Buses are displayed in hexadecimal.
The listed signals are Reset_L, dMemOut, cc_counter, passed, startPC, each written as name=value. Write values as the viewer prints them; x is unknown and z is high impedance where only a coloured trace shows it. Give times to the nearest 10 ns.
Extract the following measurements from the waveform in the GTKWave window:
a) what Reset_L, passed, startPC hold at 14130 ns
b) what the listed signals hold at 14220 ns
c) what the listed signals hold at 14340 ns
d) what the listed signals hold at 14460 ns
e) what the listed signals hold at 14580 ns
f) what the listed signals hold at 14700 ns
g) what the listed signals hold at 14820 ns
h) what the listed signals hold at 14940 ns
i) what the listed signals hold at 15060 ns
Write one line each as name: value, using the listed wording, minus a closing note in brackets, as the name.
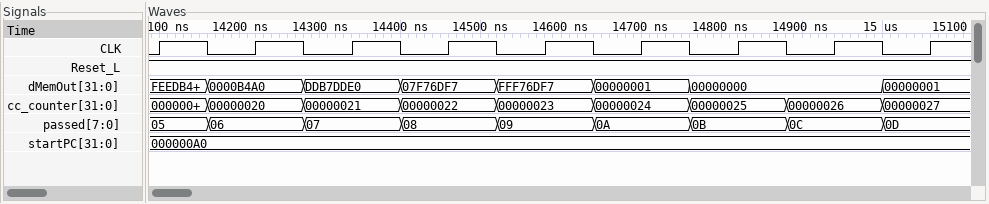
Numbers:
what Reset_L, passed, startPC hold at 14130 ns: Reset_L=1, passed=05, startPC=000000A0
what the listed signals hold at 14220 ns: Reset_L=1, dMemOut=0000B4A0, cc_counter=00000020, passed=06, startPC=000000A0
what the listed signals hold at 14340 ns: Reset_L=1, dMemOut=DDB7DDE0, cc_counter=00000021, passed=07, startPC=000000A0
what the listed signals hold at 14460 ns: Reset_L=1, dMemOut=07F76DF7, cc_counter=00000022, passed=08, startPC=000000A0
what the listed signals hold at 14580 ns: Reset_L=1, dMemOut=FFF76DF7, cc_counter=00000023, passed=09, startPC=000000A0
what the listed signals hold at 14700 ns: Reset_L=1, dMemOut=00000001, cc_counter=00000024, passed=0A, startPC=000000A0
what the listed signals hold at 14820 ns: Reset_L=1, dMemOut=00000000, cc_counter=00000025, passed=0B, startPC=000000A0
what the listed signals hold at 14940 ns: Reset_L=1, dMemOut=00000000, cc_counter=00000026, passed=0C, startPC=000000A0
what the listed signals hold at 15060 ns: Reset_L=1, dMemOut=00000001, cc_counter=00000027, passed=0D, startPC=000000A0
